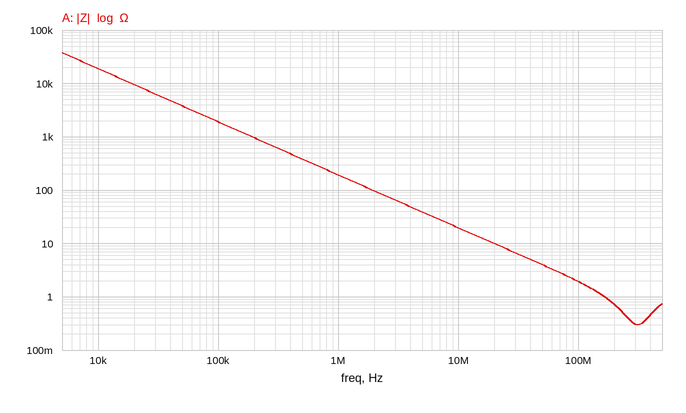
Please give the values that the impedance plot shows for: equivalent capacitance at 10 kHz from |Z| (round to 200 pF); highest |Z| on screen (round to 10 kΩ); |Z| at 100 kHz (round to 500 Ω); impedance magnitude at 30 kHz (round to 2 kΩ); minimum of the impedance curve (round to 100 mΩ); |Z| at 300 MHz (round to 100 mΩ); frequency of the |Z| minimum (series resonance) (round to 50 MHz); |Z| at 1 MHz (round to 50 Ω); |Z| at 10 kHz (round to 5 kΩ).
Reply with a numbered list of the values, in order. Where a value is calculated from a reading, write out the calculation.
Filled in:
1. C = 1/(2π × 10 kHz × 20 kΩ) ≈ 796 pF, so 800 pF to the nearest 200 pF
2. 40 kΩ
3. 2.0 kΩ
4. 6 kΩ
5. 300 mΩ
6. 300 mΩ
7. 300 MHz
8. 200 Ω
9. 20 kΩ
